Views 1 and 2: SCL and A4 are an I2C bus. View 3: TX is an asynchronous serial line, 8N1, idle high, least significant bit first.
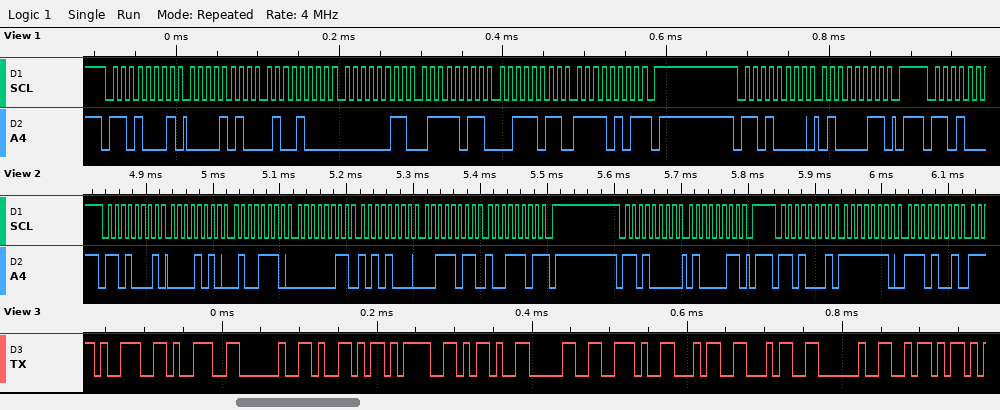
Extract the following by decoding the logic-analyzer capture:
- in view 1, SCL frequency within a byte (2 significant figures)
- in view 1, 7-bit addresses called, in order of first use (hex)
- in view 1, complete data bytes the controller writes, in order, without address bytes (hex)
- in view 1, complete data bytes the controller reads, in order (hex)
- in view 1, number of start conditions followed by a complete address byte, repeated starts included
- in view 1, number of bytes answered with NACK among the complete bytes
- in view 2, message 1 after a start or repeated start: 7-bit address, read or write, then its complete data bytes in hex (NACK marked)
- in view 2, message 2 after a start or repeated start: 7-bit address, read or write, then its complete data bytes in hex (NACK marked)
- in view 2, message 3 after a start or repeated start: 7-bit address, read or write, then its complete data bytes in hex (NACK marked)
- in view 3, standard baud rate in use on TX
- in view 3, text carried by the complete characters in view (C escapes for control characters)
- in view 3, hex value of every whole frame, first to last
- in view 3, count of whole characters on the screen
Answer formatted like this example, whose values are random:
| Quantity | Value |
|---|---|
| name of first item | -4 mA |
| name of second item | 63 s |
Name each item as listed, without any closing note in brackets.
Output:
| Quantity | Value |
|---|---|
| in view 1, SCL frequency within a byte | 100 kHz |
| in view 1, 7-bit addresses called, in order of first use | 0x68 |
| in view 1, complete data bytes the controller writes, in order, without address bytes | 43 |
| in view 1, complete data bytes the controller reads, in order | 0A 48 03 7B 3B F5 |
| in view 1, number of start conditions followed by a complete address byte, repeated starts included | 2 |
| in view 1, number of bytes answered with NACK among the complete bytes | 1 |
| in view 2, message 1 after a start or repeated start: 7-bit address, read or write, then its complete data bytes in hex | 0x68 read: 0A 4E 03 A8 3B 9D NACK |
| in view 2, message 2 after a start or repeated start: 7-bit address, read or write, then its complete data bytes in hex | 0x68 write: 43 |
| in view 2, message 3 after a start or repeated start: 7-bit address, read or write, then its complete data bytes in hex | 0x68 read: FE E9 |
| in view 3, standard baud rate in use on TX | 115200 baud |
| in view 3, text carried by the complete characters in view | "99 Y=-0.44 Z" |
| in view 3, hex value of every whole frame, first to last | 0x39 0x39 0x20 0x59 0x3D 0x2D 0x30 0x2E 0x34 0x34 0x20 0x5A |
| in view 3, count of whole characters on the screen | 12 |
